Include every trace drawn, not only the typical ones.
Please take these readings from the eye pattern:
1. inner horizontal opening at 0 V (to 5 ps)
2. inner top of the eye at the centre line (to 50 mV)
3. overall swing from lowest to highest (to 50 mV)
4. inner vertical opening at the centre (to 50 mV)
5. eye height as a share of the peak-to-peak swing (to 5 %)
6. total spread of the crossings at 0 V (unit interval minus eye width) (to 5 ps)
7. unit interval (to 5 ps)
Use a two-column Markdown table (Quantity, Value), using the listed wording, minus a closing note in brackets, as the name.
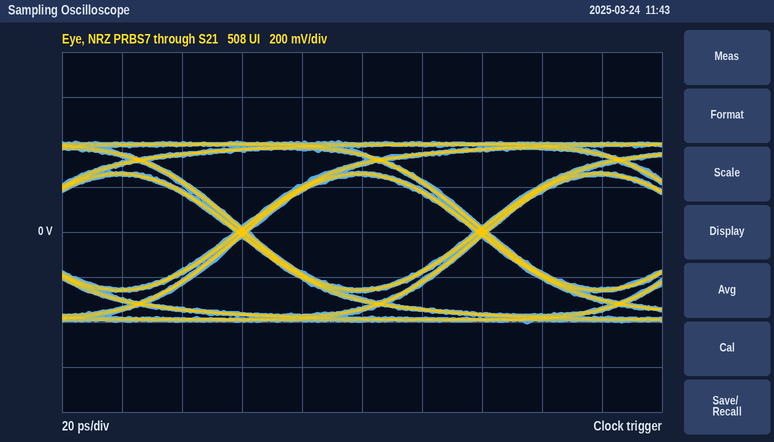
| Quantity | Value |
|---|---|
| inner horizontal opening at 0 V | 75 ps |
| inner top of the eye at the centre line | 250 mV |
| overall swing from lowest to highest | 800 mV |
| inner vertical opening at the centre | 500 mV |
| eye height as a share of the peak-to-peak swing | 60 % |
| total spread of the crossings at 0 V (unit interval minus eye width) | 5 ps |
| unit interval | 80 ps |
